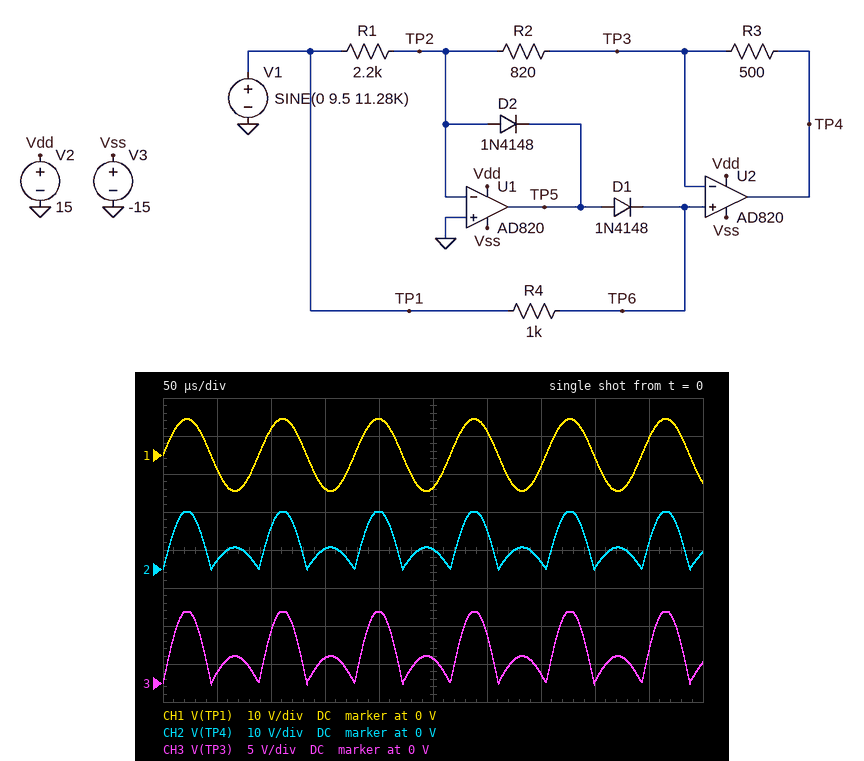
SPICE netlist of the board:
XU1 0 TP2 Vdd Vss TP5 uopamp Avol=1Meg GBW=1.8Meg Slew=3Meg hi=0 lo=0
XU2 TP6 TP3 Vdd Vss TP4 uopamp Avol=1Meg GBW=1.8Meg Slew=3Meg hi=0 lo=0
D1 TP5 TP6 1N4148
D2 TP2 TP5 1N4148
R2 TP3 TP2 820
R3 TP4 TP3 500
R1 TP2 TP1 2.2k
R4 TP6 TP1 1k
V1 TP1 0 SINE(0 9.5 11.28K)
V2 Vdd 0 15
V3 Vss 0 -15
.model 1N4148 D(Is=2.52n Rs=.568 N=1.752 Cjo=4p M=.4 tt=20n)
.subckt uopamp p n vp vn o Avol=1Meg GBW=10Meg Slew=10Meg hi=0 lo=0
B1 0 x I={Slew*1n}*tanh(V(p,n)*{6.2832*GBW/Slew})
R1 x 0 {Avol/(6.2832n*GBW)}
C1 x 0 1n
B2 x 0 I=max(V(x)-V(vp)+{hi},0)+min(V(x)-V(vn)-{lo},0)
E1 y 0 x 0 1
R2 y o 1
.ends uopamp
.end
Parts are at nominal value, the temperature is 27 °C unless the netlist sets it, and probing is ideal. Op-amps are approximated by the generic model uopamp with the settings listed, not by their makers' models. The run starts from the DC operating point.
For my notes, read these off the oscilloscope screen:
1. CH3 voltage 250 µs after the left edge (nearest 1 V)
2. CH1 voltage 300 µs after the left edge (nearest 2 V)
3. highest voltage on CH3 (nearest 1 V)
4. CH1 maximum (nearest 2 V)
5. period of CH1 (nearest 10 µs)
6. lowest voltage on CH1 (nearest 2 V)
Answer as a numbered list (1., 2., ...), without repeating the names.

1. 3 V
2. 6 V
3. 9 V
4. 10 V
5. 90 µs
6. -10 V
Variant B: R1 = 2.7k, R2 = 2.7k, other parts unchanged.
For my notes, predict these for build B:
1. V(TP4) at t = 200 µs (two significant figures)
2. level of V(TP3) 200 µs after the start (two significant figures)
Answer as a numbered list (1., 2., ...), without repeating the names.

1. 11 V
2. 9.5 V
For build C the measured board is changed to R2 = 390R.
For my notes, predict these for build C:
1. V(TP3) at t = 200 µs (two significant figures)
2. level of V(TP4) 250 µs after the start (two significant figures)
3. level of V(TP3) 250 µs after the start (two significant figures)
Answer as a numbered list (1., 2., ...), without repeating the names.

1. 6.6 V
2. 3.5 V
3. 1.5 V
